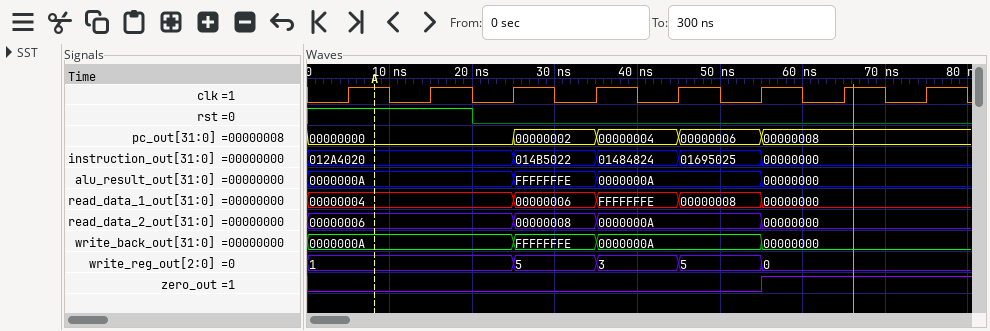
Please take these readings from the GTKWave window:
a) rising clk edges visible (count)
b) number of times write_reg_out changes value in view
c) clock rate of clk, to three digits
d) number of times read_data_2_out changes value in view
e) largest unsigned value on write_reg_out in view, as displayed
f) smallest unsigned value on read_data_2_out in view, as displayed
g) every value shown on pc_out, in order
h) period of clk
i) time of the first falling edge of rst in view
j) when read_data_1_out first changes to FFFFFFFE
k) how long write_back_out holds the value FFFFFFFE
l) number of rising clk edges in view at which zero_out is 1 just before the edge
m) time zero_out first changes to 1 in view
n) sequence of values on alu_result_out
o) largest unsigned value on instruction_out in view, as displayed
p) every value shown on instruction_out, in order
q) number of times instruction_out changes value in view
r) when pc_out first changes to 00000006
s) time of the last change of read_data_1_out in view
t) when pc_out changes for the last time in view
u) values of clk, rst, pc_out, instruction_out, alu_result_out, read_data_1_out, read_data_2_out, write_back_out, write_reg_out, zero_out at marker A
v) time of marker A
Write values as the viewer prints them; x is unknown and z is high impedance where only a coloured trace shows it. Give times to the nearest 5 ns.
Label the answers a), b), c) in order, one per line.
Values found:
a) 8
b) 4
c) 100 MHz
d) 3
e) 5
f) 00000000
g) 00000000, 00000002, 00000004, 00000006, 00000008
h) 10 ns
i) 20 ns
j) 35 ns
k) 10 ns
l) 2
m) 55 ns
n) 0000000A, FFFFFFFE, 0000000A, 00000000
o) 01695025
p) 012A4020, 014B5022, 01484824, 01695025, 00000000
q) 4
r) 45 ns
s) 55 ns
t) 55 ns
u) clk=1, rst=1, pc_out=00000000, instruction_out=012A4020, alu_result_out=0000000A, read_data_1_out=00000004, read_data_2_out=00000006, write_back_out=0000000A, write_reg_out=1, zero_out=0
v) 10 ns
